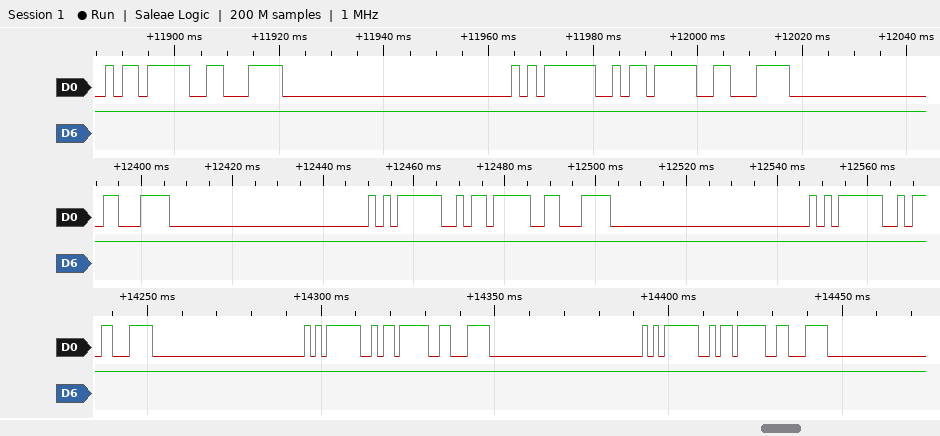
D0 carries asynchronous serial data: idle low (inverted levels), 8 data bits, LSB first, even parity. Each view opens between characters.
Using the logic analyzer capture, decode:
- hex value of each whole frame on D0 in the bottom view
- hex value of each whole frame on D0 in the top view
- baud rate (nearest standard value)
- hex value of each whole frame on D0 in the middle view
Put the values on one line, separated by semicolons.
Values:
0E, 05, 09, 0E, 05, 09, 0E; 09, 0E, 05, 09, 0E; 600 baud; 0E, 05, 09, 0E, 05
